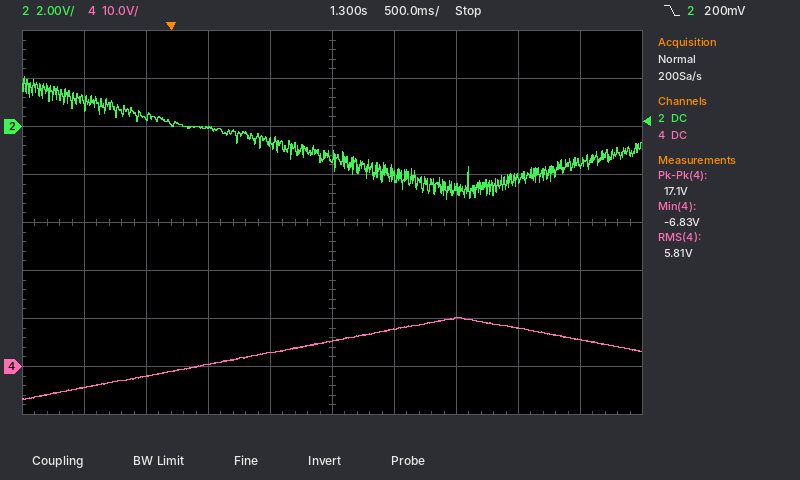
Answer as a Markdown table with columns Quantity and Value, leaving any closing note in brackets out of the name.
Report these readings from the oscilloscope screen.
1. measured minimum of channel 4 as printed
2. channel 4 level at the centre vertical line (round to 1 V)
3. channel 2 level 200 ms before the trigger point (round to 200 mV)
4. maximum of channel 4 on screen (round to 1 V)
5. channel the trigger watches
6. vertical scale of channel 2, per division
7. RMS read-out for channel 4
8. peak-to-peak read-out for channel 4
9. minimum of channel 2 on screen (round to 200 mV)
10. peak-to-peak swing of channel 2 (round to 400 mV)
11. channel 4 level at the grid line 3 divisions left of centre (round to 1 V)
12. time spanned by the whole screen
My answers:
| Quantity | Value |
|---|---|
| measured minimum of channel 4 as printed | -6.83 V |
| channel 4 level at the centre vertical line | 5 V |
| channel 2 level 200 ms before the trigger point | 400 mV |
| maximum of channel 4 on screen | 10 V |
| channel the trigger watches | channel 2 |
| vertical scale of channel 2, per division | 2 V |
| RMS read-out for channel 4 | 5.81 V |
| peak-to-peak read-out for channel 4 | 17.1 V |
| minimum of channel 2 on screen | -3.0 V |
| peak-to-peak swing of channel 2 | 5.2 V |
| channel 4 level at the grid line 3 divisions left of centre | -2 V |
| time spanned by the whole screen | 5 s |
